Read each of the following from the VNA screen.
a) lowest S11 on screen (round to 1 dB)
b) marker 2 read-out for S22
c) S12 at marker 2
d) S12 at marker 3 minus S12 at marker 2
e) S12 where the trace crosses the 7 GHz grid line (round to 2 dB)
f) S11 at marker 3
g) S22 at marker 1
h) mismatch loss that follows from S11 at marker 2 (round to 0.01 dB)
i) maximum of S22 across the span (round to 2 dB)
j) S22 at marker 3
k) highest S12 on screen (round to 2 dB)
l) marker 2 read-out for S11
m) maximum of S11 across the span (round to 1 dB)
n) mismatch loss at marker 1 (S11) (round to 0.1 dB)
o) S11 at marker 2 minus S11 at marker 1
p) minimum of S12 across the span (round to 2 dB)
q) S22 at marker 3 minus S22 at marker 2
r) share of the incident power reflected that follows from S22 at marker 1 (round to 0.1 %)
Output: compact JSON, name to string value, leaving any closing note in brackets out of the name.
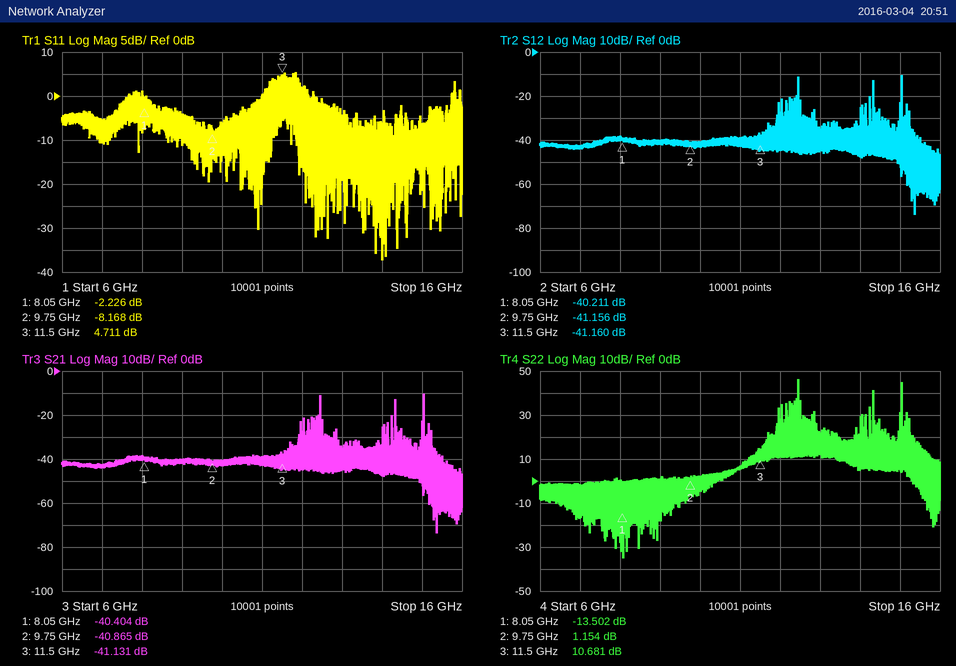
{"lowest S11 on screen": "-37 dB", "marker 2 read-out for S22": "1.154 dB", "S12 at marker 2": "-41.156 dB", "S12 at marker 3 minus S12 at marker 2": "-0.004 dB", "S12 where the trace crosses the 7 GHz grid line": "-44 dB", "S11 at marker 3": "4.711 dB", "S22 at marker 1": "-13.502 dB", "mismatch loss that follows from S11 at marker 2": "0.72 dB", "maximum of S22 across the span": "46 dB", "S22 at marker 3": "10.681 dB", "highest S12 on screen": "-10 dB", "marker 2 read-out for S11": "-8.168 dB", "maximum of S11 across the span": "5 dB", "mismatch loss at marker 1 (S11)": "4.0 dB", "S11 at marker 2 minus S11 at marker 1": "-5.942 dB", "minimum of S12 across the span": "-74 dB", "S22 at marker 3 minus S22 at marker 2": "9.527 dB", "share of the incident power reflected that follows from S22 at marker 1": "4.5 %"}
